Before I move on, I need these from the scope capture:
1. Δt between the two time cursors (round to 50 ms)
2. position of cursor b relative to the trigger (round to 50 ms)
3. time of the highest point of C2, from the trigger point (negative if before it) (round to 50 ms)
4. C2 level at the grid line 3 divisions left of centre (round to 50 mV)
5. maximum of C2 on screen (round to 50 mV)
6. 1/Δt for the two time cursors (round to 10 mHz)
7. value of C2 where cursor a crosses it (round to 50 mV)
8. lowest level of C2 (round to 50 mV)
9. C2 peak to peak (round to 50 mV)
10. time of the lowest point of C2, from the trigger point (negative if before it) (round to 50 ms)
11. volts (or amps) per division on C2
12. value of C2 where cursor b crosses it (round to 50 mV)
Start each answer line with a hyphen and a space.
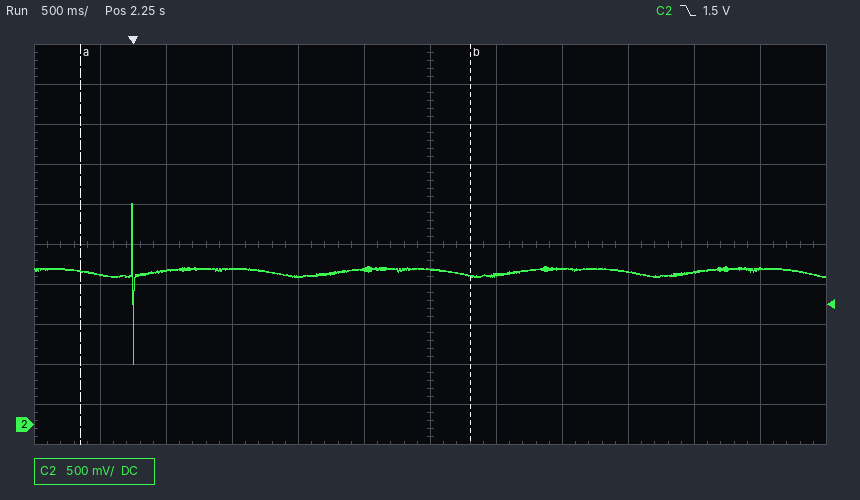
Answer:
- 2.95 s
- +2.55 s
- 0 ms
- 1.95 V
- 2.75 V
- 340 mHz
- 1.90 V
- 750 mV
- 2.00 V
- 0 ms
- 500 mV
- 1.85 V
